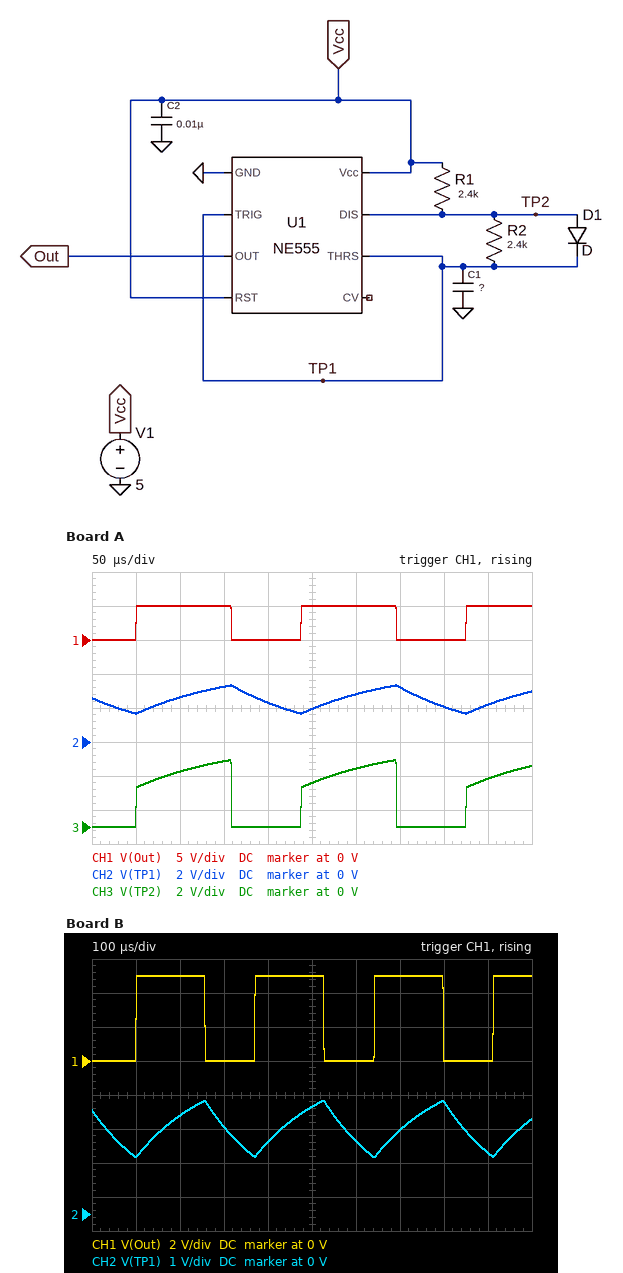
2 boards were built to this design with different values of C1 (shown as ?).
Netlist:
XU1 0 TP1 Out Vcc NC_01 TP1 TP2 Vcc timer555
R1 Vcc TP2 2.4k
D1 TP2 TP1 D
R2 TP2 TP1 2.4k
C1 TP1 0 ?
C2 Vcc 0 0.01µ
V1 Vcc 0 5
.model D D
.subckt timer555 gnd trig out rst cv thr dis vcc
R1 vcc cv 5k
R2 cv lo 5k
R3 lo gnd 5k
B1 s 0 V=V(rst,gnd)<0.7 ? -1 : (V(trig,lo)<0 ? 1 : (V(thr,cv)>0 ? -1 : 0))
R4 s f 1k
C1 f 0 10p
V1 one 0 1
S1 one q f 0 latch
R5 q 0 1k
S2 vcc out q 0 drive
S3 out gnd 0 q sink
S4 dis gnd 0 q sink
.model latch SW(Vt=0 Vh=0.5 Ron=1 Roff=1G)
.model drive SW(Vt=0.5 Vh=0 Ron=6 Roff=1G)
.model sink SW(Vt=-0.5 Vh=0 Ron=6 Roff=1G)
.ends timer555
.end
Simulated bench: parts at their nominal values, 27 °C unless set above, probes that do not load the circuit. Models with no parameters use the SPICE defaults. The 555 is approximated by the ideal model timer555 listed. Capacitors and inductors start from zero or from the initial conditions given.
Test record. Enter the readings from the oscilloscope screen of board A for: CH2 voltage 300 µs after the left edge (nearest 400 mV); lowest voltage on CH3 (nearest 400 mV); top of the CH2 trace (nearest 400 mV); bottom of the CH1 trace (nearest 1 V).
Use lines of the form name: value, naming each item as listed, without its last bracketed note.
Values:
CH2 voltage 300 µs after the left edge: 2.8 V
lowest voltage on CH3: 0 V
top of the CH2 trace: 3.2 V
bottom of the CH1 trace: 0 V
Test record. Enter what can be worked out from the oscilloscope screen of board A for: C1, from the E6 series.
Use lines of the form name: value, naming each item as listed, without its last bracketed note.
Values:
C1, from the E6 series: 47 nF
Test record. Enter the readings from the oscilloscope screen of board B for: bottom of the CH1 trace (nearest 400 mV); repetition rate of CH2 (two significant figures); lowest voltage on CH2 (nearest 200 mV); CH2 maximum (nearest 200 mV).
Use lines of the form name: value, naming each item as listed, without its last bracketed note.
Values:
bottom of the CH1 trace: 0 V
repetition rate of CH2: 3.7 kHz
lowest voltage on CH2: 1.6 V
CH2 maximum: 3.4 V
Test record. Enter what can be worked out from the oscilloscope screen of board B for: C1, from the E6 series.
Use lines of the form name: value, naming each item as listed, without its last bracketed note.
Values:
C1, from the E6 series: 68 nF
